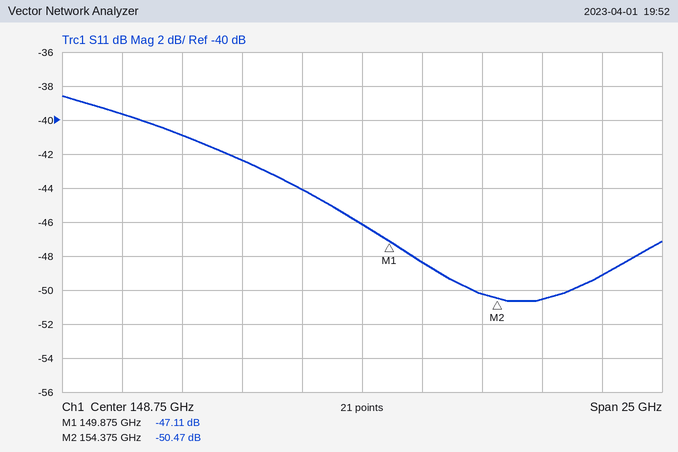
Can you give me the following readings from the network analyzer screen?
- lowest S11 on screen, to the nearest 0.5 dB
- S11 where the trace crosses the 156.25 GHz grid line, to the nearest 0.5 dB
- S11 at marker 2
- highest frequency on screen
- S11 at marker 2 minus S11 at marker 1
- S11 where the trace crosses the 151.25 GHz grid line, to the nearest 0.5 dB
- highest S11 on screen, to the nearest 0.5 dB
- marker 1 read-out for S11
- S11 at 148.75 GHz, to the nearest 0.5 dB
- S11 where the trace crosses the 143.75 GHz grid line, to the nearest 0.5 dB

-50.5 dB
-50.5 dB
-50.47 dB
161.25 GHz
-3.36 dB
-48.5 dB
-38.5 dB
-47.11 dB
-46.0 dB
-42.5 dB
